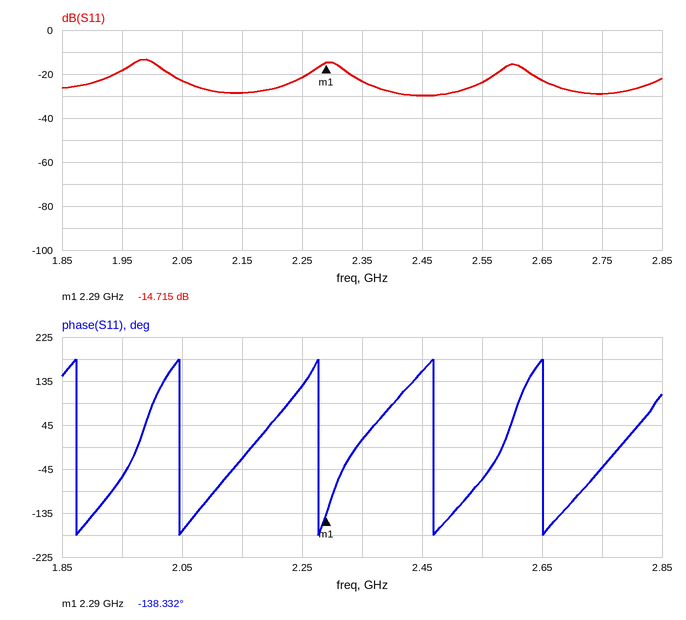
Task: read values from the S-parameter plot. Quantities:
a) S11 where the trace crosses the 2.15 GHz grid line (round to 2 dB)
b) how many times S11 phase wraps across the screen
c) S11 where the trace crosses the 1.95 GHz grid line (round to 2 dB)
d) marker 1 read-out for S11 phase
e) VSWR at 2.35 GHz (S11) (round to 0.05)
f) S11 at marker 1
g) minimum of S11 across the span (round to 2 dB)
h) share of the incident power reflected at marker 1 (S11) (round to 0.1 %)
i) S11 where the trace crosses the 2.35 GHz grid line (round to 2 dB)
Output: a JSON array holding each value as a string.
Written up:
["-28 dB", "5", "-18 dB", "-138.332°", "1.15", "-14.715 dB", "-30 dB", "3.4 %", "-24 dB"]
